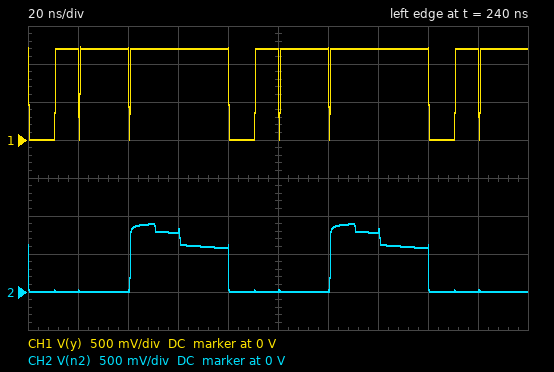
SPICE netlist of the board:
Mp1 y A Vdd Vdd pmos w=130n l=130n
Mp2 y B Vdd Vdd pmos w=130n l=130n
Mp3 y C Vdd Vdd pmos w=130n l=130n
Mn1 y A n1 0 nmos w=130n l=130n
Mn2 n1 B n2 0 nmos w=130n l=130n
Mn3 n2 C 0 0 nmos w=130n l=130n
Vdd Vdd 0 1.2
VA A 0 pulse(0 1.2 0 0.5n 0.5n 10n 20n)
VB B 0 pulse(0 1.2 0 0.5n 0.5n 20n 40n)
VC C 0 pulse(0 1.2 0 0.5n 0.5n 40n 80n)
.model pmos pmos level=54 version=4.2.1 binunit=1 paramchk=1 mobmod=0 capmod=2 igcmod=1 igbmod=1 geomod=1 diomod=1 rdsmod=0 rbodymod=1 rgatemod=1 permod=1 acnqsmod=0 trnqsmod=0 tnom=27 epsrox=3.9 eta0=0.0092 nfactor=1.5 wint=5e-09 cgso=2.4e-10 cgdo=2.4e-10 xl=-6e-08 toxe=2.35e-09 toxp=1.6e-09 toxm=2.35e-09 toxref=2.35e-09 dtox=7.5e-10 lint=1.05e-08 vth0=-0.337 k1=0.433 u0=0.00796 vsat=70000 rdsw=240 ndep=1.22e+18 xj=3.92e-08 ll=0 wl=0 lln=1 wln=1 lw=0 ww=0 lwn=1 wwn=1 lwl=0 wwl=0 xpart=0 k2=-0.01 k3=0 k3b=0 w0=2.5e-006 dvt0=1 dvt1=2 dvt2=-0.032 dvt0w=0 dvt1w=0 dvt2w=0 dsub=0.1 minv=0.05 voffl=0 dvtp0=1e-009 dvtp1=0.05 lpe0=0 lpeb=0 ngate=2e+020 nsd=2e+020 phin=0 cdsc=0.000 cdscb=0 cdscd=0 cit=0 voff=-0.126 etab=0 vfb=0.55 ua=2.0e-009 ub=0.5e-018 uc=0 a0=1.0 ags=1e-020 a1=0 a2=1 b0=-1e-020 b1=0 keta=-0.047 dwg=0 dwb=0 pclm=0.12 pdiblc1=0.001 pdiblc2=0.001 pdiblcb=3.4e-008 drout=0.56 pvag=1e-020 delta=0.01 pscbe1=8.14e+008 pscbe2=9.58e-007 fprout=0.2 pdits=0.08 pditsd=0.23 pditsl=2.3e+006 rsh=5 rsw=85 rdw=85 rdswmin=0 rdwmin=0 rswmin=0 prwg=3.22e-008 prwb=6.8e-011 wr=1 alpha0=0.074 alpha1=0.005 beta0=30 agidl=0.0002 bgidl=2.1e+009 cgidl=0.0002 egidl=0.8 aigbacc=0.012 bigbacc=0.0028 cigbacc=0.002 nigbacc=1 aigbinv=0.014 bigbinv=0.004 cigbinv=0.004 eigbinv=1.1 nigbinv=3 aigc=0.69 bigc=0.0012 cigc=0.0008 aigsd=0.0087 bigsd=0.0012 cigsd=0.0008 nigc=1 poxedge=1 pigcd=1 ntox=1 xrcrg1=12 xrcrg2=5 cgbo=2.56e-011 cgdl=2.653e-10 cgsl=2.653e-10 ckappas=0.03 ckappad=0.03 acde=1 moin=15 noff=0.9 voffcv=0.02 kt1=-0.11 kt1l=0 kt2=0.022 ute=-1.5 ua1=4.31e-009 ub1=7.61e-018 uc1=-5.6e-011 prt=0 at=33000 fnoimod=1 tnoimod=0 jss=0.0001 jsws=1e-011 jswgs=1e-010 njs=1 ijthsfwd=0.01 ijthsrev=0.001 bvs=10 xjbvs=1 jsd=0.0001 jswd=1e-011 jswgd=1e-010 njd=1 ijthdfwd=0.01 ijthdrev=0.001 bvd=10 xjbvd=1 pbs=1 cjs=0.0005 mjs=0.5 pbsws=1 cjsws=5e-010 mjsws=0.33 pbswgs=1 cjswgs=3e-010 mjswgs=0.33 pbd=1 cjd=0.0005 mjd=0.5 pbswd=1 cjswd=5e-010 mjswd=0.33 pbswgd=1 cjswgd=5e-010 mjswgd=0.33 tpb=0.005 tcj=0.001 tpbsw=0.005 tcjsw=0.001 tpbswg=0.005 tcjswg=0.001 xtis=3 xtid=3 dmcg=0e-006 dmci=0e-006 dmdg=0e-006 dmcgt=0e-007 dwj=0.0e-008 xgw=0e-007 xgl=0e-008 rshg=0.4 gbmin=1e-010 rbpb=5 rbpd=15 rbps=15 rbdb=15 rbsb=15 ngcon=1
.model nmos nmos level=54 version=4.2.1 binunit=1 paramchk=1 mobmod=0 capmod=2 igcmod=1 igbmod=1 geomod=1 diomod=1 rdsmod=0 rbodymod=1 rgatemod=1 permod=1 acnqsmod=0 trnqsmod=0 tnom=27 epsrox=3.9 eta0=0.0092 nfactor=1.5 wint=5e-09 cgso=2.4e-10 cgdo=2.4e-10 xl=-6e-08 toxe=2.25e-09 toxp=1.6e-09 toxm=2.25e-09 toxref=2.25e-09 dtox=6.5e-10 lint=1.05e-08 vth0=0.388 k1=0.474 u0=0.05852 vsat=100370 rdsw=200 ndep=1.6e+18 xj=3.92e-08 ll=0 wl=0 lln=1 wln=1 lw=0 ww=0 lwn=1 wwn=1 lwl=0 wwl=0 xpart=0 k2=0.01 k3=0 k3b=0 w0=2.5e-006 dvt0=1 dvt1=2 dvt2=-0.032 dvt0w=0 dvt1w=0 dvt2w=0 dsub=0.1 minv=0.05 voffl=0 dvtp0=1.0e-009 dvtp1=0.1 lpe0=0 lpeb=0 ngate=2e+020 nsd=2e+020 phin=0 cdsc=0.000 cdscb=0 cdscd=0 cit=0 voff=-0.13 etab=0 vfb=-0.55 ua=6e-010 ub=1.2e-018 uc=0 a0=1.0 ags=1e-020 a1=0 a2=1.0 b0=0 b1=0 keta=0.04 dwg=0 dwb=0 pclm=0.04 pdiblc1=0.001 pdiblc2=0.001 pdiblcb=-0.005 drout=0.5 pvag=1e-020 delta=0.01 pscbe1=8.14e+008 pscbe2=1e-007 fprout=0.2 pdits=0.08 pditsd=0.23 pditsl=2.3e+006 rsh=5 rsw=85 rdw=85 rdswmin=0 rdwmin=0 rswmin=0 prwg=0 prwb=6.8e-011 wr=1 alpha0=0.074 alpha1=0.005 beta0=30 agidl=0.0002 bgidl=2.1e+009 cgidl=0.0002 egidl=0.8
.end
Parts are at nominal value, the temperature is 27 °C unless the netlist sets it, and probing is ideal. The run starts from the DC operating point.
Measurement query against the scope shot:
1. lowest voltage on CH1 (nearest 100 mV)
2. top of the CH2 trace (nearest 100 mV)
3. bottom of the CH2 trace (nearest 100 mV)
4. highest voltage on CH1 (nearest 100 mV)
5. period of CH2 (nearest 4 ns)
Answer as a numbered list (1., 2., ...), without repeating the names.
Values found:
1. 0 V
2. 900 mV
3. 0 V
4. 1.2 V
5. 80 ns
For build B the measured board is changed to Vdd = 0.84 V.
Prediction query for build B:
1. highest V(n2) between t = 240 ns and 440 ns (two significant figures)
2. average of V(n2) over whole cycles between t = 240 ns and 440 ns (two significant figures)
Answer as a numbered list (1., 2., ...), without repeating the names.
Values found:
1. 840 mV
2. 330 mV
